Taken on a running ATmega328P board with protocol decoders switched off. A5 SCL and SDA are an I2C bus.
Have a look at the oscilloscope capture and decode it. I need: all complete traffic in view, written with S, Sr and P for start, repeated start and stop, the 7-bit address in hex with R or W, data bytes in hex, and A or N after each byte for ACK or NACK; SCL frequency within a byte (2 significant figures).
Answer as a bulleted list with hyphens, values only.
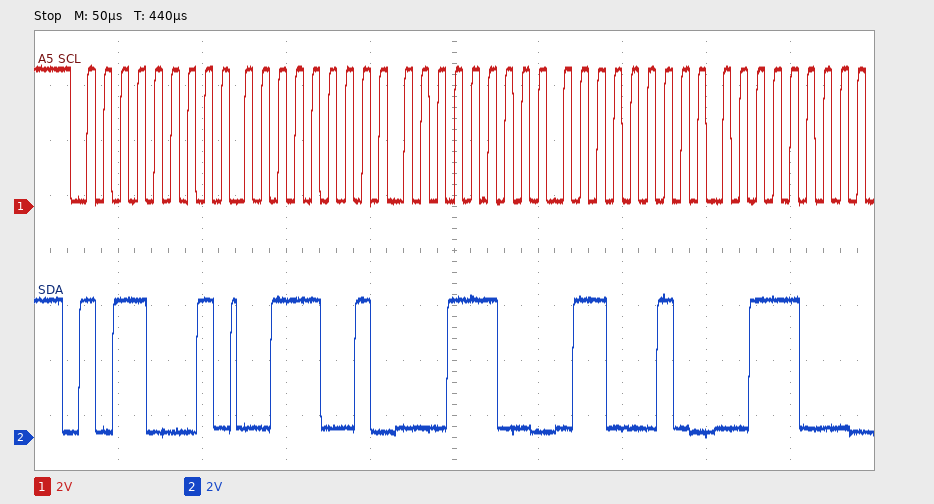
- S 58R A 39 A 1C A 62 A 38 A
- 100 kHz
